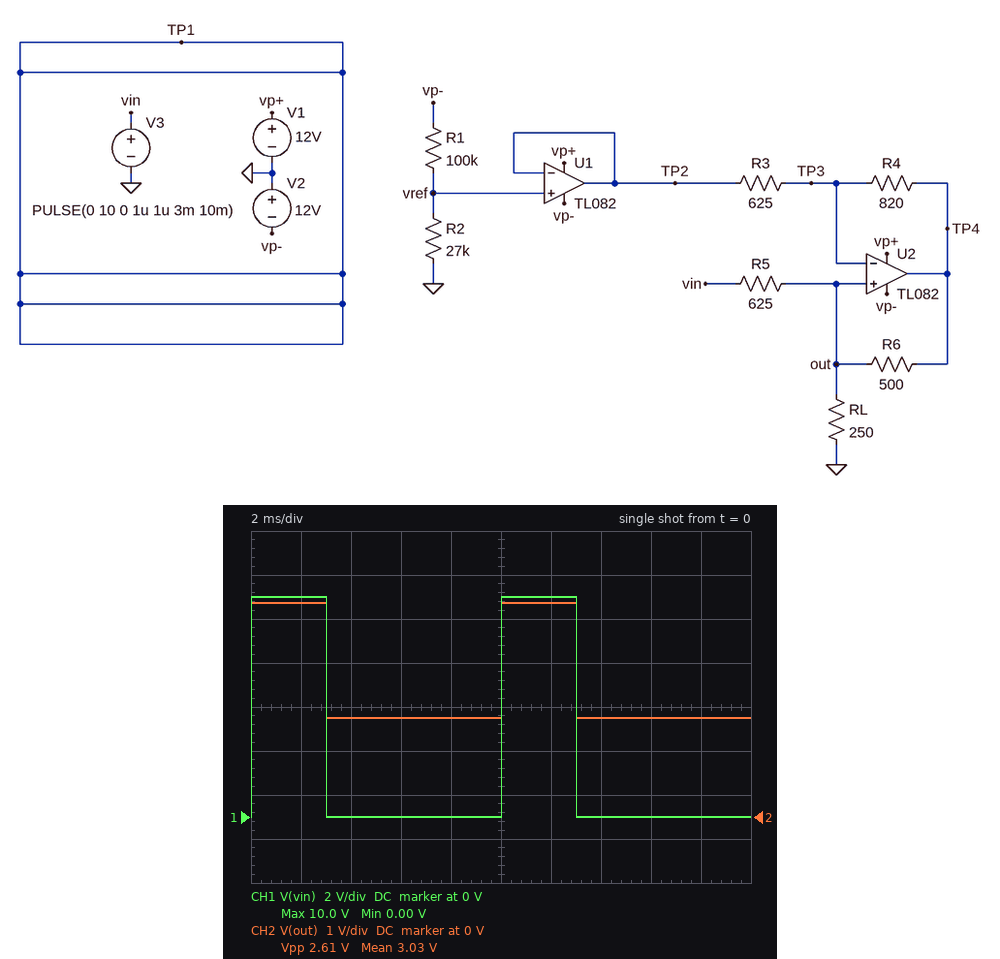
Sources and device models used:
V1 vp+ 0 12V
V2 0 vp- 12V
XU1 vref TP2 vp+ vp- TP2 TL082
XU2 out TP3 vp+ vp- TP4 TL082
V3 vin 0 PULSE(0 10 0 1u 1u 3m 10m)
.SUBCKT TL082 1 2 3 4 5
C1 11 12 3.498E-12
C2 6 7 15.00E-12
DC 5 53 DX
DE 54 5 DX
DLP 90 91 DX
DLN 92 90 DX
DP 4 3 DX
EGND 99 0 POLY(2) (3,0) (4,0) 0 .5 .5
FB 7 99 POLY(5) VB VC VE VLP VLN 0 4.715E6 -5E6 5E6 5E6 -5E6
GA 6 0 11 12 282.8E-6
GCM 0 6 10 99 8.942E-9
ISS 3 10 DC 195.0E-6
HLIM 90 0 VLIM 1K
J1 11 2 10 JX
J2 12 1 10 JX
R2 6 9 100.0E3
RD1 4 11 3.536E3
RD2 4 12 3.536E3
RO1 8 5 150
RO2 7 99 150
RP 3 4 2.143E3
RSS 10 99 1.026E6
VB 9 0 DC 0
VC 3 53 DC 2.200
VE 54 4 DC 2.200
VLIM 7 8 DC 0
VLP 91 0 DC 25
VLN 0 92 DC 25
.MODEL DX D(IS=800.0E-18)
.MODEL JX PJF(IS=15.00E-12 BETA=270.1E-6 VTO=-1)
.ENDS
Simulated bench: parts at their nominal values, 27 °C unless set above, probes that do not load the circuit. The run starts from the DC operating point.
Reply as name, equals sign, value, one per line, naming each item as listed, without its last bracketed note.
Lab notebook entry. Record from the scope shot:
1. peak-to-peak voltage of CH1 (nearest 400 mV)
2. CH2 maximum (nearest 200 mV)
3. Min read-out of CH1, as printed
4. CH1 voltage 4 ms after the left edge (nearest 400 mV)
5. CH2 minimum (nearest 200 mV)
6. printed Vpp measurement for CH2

peak-to-peak voltage of CH1 = 10.0 V
CH2 maximum = 4.8 V
Min read-out of CH1, as printed = 0.00 V
CH1 voltage 4 ms after the left edge = 0 V
CH2 minimum = 2.2 V
printed Vpp measurement for CH2 = 2.61 V
